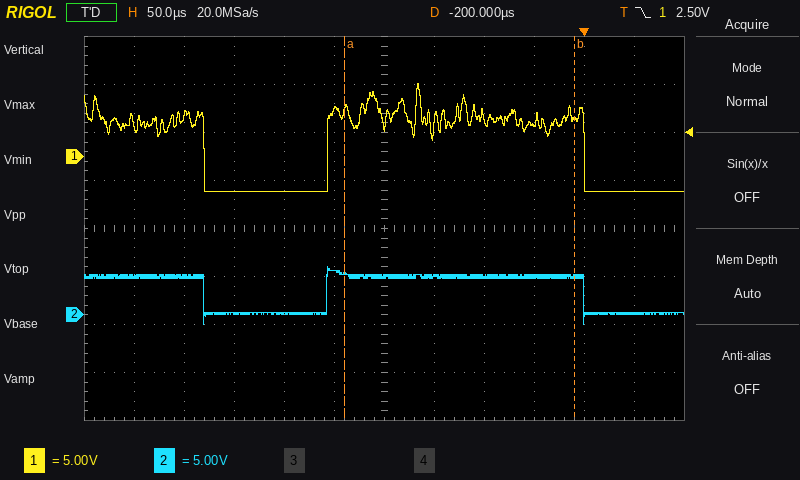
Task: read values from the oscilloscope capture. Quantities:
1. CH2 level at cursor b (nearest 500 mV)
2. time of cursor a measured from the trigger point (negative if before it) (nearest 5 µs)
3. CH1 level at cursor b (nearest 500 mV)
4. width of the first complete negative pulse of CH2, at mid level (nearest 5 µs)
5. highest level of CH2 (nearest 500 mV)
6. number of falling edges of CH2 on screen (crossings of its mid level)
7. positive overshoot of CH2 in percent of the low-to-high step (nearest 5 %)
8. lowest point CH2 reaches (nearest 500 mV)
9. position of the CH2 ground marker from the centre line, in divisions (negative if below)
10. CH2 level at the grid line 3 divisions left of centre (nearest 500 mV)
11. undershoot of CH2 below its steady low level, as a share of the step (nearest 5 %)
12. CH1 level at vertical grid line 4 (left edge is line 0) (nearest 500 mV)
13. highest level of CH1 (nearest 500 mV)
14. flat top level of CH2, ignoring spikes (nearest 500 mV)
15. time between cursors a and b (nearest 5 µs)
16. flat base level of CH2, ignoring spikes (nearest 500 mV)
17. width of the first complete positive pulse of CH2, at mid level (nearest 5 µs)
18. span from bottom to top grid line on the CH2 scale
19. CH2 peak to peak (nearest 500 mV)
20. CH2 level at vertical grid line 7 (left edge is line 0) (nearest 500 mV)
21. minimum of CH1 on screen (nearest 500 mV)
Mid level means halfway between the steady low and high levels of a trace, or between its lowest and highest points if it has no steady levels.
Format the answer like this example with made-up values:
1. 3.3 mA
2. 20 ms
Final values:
1. 4.0 V
2. -240 µs
3. 4.0 V
4. 125 µs
5. 5.0 V
6. 2
7. 25 %
8. -1.0 V
9. -1.8 div
10. 0.0 V
11. 30 %
12. -3.5 V
13. 7.5 V
14. 4.0 V
15. 230 µs
16. 0.0 V
17. 255 µs
18. 40 V
19. 6.0 V
20. 4.0 V
21. -3.5 V
